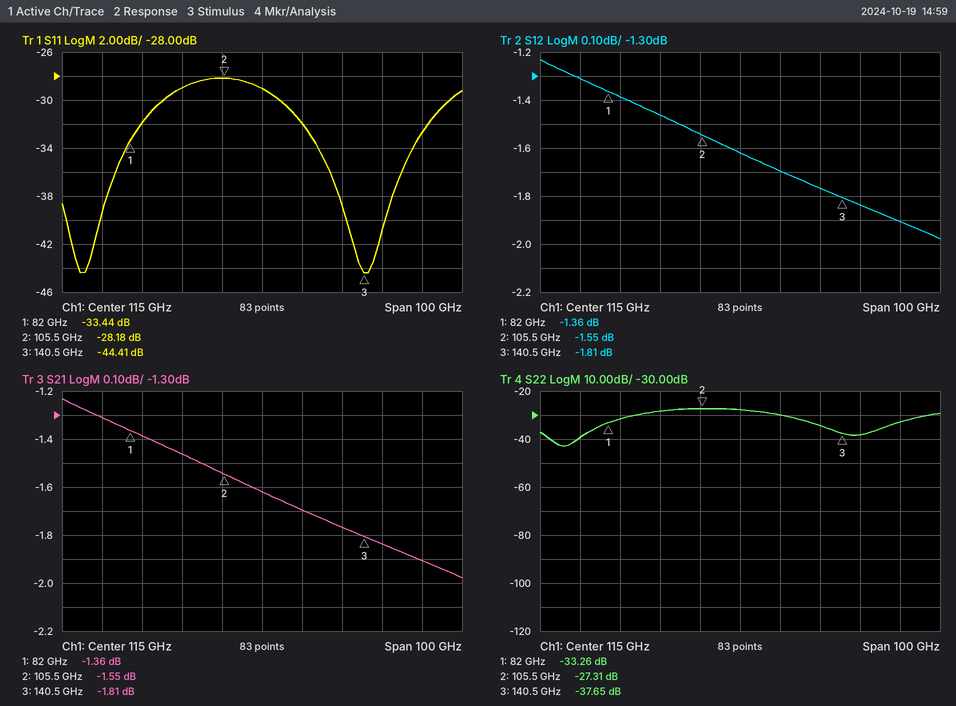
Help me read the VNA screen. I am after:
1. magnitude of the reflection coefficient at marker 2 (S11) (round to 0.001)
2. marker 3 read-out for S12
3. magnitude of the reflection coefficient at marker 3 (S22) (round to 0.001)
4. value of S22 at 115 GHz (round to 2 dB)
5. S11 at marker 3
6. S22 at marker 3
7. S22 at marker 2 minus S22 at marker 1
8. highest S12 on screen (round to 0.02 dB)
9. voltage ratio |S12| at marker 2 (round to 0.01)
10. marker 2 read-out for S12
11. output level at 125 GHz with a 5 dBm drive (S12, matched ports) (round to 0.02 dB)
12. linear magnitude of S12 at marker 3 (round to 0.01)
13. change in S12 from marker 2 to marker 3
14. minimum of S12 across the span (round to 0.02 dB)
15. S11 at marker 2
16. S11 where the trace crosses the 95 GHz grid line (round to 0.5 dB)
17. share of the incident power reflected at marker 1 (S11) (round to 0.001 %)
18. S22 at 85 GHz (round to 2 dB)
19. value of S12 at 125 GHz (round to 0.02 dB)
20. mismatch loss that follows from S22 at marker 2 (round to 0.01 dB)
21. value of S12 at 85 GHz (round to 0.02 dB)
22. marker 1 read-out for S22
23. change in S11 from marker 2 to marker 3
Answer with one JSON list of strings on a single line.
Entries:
["0.039", "-1.81 dB", "0.013", "-28 dB", "-44.41 dB", "-37.65 dB", "5.95 dB", "-1.24 dB", "0.84", "-1.55 dB", "3.30 dBm", "0.81", "-0.26 dB", "-1.98 dB", "-28.18 dB", "-29.0 dB", "0.045 %", "-32 dB", "-1.70 dB", "0.01 dB", "-1.38 dB", "-33.26 dB", "-16.23 dB"]
